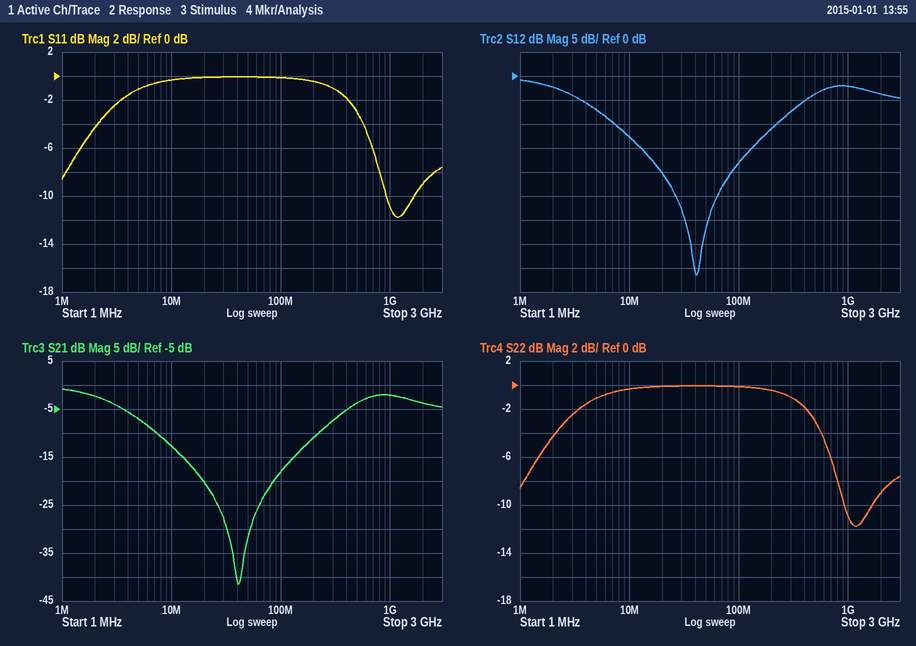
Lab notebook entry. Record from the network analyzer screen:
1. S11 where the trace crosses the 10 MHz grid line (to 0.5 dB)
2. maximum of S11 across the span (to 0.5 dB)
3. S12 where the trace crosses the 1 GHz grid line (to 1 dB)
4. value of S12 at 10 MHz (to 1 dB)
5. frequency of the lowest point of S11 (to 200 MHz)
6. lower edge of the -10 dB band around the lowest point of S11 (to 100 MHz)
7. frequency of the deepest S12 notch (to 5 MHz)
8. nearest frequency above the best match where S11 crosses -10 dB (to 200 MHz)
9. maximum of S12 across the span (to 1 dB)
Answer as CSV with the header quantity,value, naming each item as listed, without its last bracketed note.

quantity,value
S11 where the trace crosses the 10 MHz grid line,-0.5 dB
maximum of S11 across the span,0.0 dB
S12 where the trace crosses the 1 GHz grid line,-2 dB
value of S12 at 10 MHz,-13 dB
frequency of the lowest point of S11,1.2 GHz
lower edge of the -10 dB band around the lowest point of S11,900 MHz
frequency of the deepest S12 notch,40 MHz
nearest frequency above the best match where S11 crosses -10 dB,1.6 GHz
maximum of S12 across the span,-1 dB
